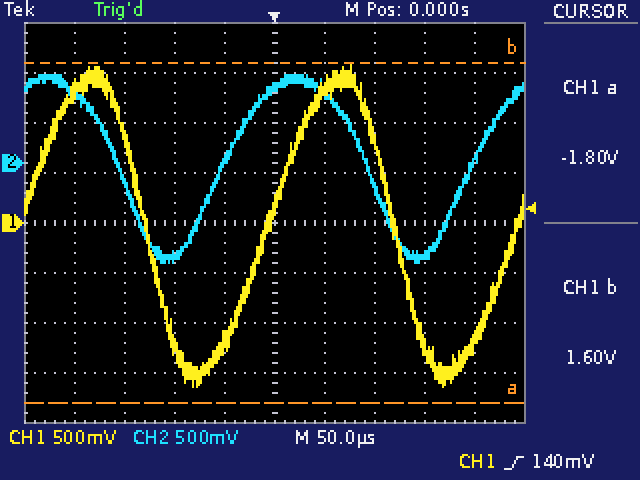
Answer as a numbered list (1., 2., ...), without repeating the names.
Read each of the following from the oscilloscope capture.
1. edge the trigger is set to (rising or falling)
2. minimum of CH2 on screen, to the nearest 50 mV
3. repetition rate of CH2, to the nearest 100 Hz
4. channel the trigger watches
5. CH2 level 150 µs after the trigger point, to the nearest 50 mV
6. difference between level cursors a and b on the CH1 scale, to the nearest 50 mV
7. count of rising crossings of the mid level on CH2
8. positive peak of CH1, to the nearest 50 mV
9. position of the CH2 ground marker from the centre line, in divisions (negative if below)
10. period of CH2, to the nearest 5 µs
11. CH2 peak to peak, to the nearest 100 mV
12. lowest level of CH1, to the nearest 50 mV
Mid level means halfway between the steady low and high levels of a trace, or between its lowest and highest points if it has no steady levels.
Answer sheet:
1. rising
2. -1.00 V
3. 4.0 kHz
4. CH1
5. -900 mV
6. 3.40 V
7. 2
8. 1.60 V
9. +1.2 div
10. 250 µs
11. 1.90 V
12. -1.65 V
